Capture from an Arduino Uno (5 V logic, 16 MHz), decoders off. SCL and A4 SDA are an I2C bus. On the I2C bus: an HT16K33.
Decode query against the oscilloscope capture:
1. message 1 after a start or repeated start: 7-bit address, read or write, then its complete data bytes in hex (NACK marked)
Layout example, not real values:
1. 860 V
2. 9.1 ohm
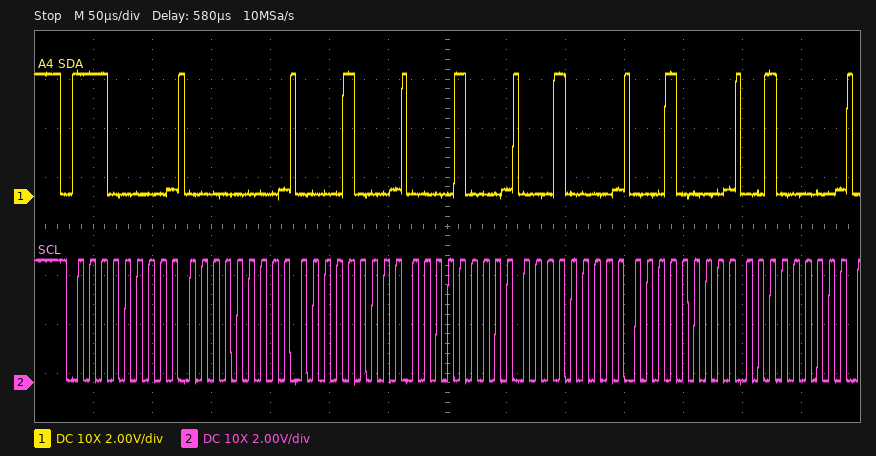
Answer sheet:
1. 0x70 write: 00 08 08 10 10 20
